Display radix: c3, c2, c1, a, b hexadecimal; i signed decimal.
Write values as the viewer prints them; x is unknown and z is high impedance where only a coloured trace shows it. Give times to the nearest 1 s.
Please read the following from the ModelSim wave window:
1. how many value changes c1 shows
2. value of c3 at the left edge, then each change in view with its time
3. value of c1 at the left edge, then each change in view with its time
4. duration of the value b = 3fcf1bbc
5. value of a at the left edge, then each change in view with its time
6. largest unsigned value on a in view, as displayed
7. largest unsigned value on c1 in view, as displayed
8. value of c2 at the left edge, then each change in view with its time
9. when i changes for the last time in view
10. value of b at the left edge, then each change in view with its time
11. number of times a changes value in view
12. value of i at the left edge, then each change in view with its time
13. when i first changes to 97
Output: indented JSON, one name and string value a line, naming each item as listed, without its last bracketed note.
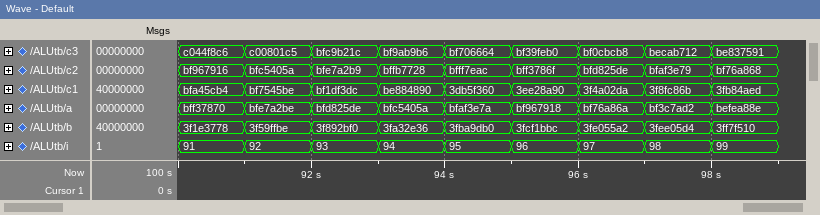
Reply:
{
  "how many value changes c1 shows": "8",
  "value of c3 at the left edge, then each change in view with its time": "c044f8c6, c00801c5 at 91 s, bfc9b21c at 92 s, bf9ab9b6 at 93 s, bf706664 at 94 s, bf39feb0 at 95 s, bf0cbcb8 at 96 s, becab712 at 97 s, be837591 at 98 s",
  "value of c1 at the left edge, then each change in view with its time": "bfa45cb4, bf7545be at 91 s, bf1df3dc at 92 s, be884890 at 93 s, 3db5f360 at 94 s, 3ee28a90 at 95 s, 3f4a02da at 96 s, 3f8fc86b at 97 s, 3fb84aed at 98 s",
  "duration of the value b = 3fcf1bbc": "1 s",
  "value of a at the left edge, then each change in view with its time": "bff37870, bfe7a2be at 91 s, bfd825de at 92 s, bfc5405a at 93 s, bfaf3e7a at 94 s, bf967918 at 95 s, bf76a86a at 96 s, bf3c7ad2 at 97 s, befea88e at 98 s",
  "largest unsigned value on a in view, as displayed": "bff37870",
  "largest unsigned value on c1 in view, as displayed": "bfa45cb4",
  "value of c2 at the left edge, then each change in view with its time": "bf967916, bfc5405a at 91 s, bfe7a2b9 at 92 s, bffb7728 at 93 s, bfff7eac at 94 s, bff3786f at 95 s, bfd825de at 96 s, bfaf3e79 at 97 s, bf76a868 at 98 s",
  "when i changes for the last time in view": "98 s",
  "value of b at the left edge, then each change in view with its time": "3f1e3778, 3f59ffbe at 91 s, 3f892bf0 at 92 s, 3fa32e36 at 93 s, 3fba9db0 at 94 s, 3fcf1bbc at 95 s, 3fe055a2 at 96 s, 3fee05d4 at 97 s, 3ff7f510 at 98 s",
  "number of times a changes value in view": "8",
  "value of i at the left edge, then each change in view with its time": "91, 92 at 91 s, 93 at 92 s, 94 at 93 s, 95 at 94 s, 96 at 95 s, 97 at 96 s, 98 at 97 s, 99 at 98 s",
  "when i first changes to 97": "96 s"
}
